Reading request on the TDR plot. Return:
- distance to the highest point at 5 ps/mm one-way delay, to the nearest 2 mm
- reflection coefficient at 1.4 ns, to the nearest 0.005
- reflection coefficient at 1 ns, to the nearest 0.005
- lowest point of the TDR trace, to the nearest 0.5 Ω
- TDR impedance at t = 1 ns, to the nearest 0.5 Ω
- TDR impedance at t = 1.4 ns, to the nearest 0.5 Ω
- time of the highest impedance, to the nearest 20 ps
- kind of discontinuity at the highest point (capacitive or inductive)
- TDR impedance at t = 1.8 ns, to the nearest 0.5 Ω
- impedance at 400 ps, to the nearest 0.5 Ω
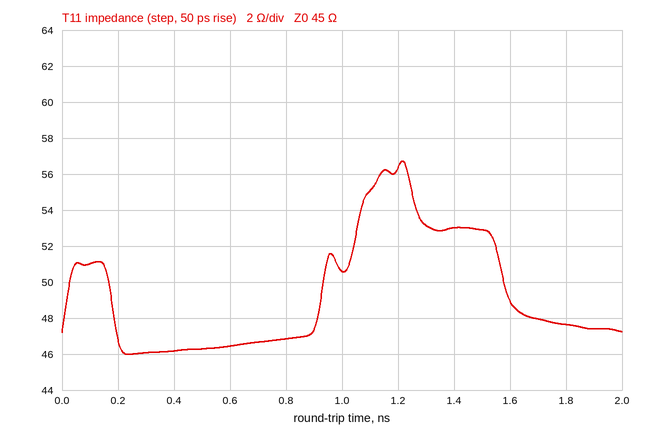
122 mm
+0.080
+0.060
46.0 Ω
50.5 Ω
53.0 Ω
1.22 ns
inductive
47.5 Ω
46.0 Ω
